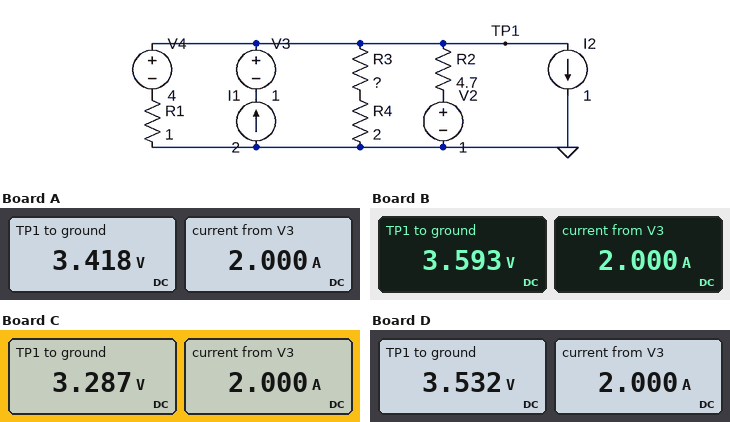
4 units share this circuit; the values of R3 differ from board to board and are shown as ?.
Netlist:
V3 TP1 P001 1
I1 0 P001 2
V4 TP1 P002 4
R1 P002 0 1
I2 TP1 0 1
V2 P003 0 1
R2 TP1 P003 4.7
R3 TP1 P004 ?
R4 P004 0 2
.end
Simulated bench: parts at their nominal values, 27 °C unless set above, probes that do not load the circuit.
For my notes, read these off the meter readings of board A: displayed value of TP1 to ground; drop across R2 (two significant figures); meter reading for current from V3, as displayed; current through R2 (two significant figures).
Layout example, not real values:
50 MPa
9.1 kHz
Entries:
3.418 V
2.4 V
2.000 A
510 mA
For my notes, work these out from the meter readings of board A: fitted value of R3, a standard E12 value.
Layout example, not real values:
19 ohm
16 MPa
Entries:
1.2 Ω
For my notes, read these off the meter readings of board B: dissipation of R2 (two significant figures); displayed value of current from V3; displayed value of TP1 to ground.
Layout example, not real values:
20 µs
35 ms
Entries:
1.4 W
2.000 A
3.593 V
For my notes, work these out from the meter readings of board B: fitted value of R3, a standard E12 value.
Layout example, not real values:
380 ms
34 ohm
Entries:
2.2 Ω
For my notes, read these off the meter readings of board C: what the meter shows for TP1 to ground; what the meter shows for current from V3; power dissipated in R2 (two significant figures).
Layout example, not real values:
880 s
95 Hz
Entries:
3.287 V
2.000 A
1.1 W
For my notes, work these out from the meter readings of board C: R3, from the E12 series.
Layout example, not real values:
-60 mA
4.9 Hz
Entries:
0.68 Ω
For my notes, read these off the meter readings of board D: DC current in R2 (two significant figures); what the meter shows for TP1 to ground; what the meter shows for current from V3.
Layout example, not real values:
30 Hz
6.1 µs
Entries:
540 mA
3.532 V
2.000 A
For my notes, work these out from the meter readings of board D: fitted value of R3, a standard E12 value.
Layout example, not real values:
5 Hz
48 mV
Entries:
1.8 Ω
